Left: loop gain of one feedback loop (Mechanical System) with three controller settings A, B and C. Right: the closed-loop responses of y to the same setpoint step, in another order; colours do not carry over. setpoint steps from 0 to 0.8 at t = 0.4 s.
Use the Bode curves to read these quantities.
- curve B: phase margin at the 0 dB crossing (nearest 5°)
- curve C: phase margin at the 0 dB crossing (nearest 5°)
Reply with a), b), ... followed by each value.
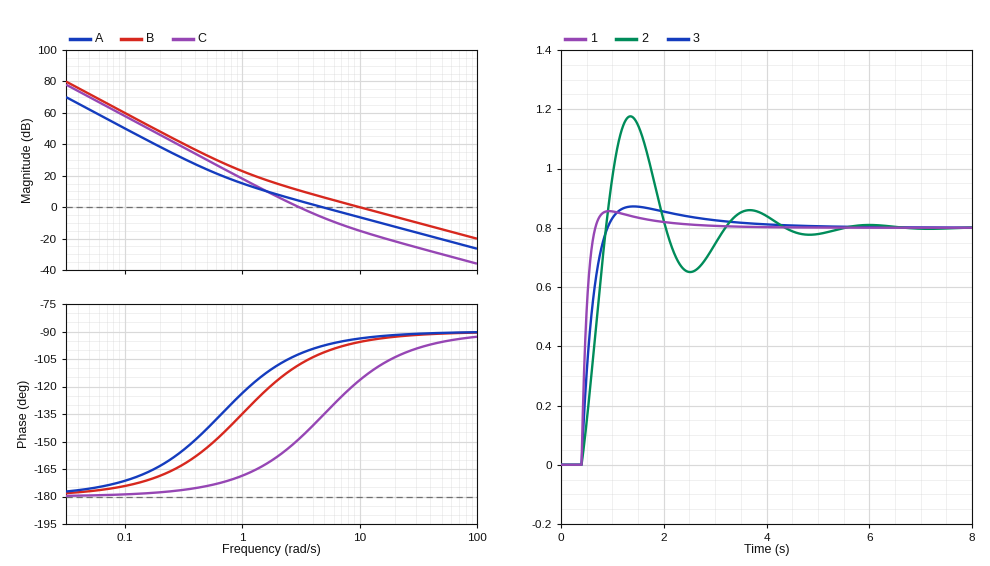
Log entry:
a) 85°
b) 30°
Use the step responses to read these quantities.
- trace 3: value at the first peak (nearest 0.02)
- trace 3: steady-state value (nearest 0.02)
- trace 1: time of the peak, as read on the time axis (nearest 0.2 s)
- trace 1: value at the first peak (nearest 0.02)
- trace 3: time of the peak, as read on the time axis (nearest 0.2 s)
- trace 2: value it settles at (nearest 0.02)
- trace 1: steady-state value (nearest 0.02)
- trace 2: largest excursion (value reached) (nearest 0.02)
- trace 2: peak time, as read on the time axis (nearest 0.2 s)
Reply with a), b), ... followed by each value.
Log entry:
a) 0.88
b) 0.80
c) 1.0 s
d) 0.86
e) 1.4 s
f) 0.80
g) 0.80
h) 1.18
i) 1.4 s
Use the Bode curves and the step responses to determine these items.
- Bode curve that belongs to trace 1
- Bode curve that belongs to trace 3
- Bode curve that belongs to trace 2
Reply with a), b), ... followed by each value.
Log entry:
a) B
b) A
c) C
